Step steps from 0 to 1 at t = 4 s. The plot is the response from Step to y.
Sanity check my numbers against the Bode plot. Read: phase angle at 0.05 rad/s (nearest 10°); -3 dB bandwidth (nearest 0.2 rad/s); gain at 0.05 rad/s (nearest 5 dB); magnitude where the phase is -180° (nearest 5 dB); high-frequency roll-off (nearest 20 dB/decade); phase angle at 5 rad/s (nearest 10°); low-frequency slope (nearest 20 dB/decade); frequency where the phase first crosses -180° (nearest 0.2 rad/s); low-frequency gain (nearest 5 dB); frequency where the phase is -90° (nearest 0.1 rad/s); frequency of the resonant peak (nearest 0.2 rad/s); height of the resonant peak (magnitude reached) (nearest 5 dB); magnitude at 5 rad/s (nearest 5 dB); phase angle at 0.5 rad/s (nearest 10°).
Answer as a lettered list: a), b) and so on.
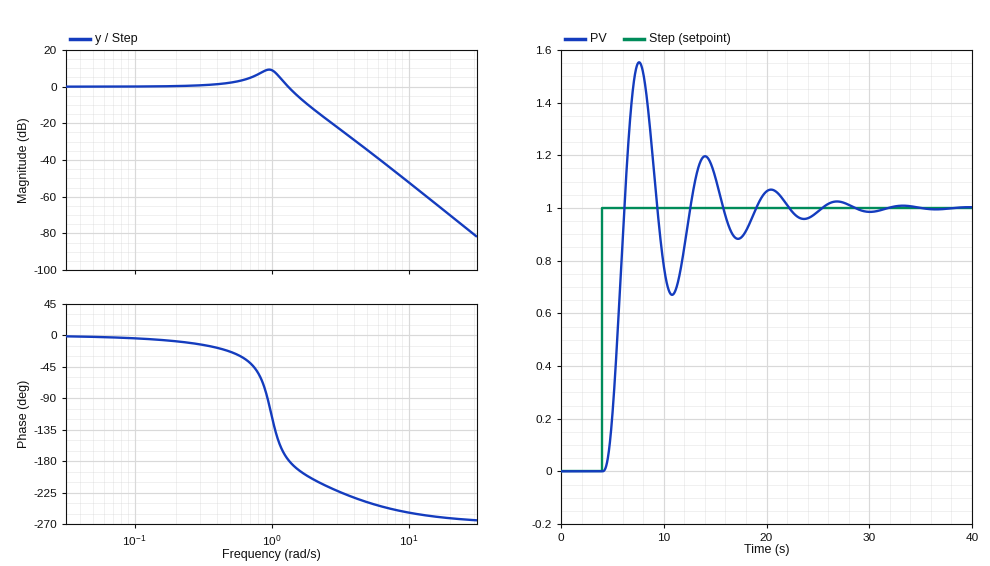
a) 0°
b) 1.4 rad/s
c) 0 dB
d) 0 dB
e) -60 dB/decade
f) -240°
g) 0 dB/decade
h) 1.4 rad/s
i) 0 dB
j) 0.9 rad/s
k) 1.0 rad/s
l) 10 dB
m) -35 dB
n) -20°
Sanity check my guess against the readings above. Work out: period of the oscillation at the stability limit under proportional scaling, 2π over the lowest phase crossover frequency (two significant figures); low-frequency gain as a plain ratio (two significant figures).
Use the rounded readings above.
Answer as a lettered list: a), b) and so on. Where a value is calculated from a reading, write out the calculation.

a) 2π / 1.4 = 4.5 s
b) 10^(0 / 20) = 1.0
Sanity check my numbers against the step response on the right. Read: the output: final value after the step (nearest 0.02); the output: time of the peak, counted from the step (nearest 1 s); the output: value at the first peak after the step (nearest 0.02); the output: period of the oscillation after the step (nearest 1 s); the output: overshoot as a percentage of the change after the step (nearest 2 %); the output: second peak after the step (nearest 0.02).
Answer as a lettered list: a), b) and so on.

a) 1.00
b) 4 s
c) 1.56
d) 6 s
e) 56 %
f) 1.20
